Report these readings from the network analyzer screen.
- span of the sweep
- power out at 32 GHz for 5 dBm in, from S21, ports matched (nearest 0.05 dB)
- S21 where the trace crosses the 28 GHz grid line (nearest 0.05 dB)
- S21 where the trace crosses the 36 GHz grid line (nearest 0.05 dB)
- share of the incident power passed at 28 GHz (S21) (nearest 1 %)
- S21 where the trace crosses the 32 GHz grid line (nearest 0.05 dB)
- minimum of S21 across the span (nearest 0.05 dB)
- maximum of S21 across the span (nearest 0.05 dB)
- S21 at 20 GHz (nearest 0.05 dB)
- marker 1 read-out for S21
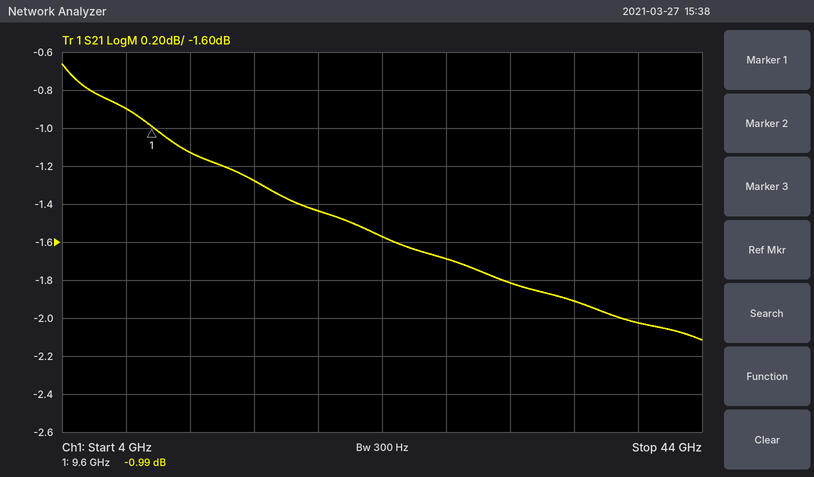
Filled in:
40 GHz
3.20 dBm
-1.70 dB
-1.90 dB
68 %
-1.80 dB
-2.10 dB
-0.65 dB
-1.45 dB
-0.99 dB
